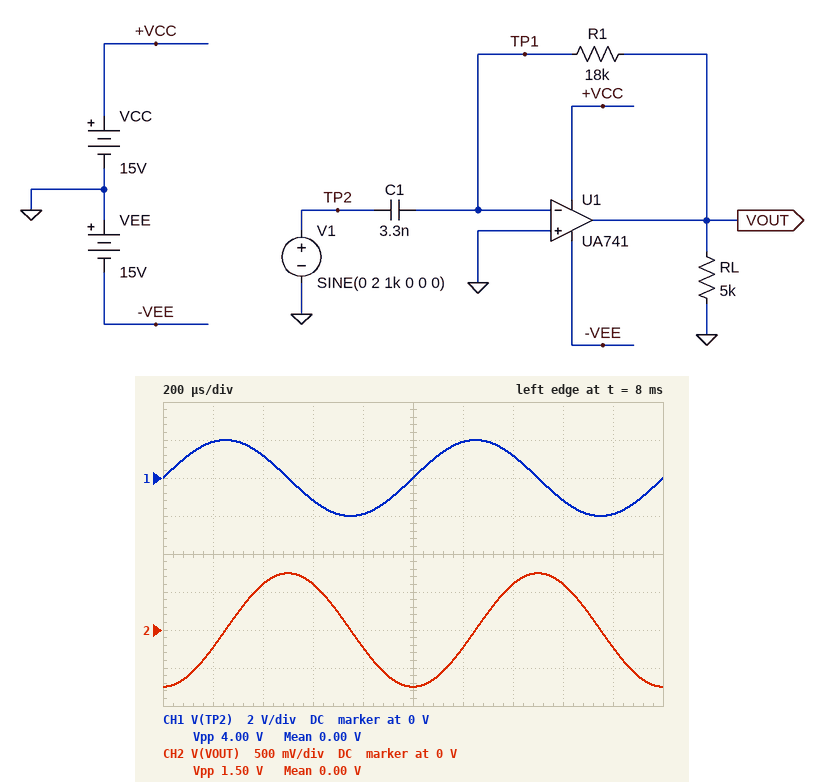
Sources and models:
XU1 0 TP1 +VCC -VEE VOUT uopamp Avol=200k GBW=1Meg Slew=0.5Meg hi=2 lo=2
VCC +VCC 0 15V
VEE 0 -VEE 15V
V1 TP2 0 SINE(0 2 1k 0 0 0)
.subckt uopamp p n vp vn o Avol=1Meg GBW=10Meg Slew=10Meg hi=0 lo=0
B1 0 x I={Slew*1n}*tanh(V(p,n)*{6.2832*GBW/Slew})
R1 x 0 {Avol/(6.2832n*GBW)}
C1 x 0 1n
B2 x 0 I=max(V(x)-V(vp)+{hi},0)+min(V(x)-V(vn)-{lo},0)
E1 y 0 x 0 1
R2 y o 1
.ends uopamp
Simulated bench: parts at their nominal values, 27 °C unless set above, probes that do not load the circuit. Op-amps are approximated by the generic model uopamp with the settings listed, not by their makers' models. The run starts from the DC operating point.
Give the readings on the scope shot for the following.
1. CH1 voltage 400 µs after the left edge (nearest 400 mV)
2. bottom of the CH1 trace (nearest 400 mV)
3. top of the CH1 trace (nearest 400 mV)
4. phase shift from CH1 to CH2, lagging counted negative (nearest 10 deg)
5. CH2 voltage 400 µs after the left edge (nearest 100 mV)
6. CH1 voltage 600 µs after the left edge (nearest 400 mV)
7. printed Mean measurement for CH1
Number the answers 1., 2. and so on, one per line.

1. 1.2 V
2. -2.0 V
3. 2.0 V
4. -90 deg
5. 600 mV
6. -1.2 V
7. 0.00 V
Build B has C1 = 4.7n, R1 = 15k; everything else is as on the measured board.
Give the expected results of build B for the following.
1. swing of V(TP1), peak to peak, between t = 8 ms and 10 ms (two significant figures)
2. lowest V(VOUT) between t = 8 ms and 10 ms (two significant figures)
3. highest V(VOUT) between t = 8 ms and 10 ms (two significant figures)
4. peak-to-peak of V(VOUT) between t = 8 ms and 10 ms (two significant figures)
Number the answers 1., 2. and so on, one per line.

1. 1.8 mV
2. -890 mV
3. 890 mV
4. 1.8 V
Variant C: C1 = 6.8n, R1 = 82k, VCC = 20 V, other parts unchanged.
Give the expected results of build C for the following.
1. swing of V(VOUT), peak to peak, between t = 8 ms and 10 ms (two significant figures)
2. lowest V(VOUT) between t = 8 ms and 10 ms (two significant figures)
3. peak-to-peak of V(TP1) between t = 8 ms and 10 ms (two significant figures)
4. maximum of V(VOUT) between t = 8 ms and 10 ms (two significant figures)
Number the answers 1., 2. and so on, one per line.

1. 14 V
2. -7.0 V
3. 14 mV
4. 7.0 V
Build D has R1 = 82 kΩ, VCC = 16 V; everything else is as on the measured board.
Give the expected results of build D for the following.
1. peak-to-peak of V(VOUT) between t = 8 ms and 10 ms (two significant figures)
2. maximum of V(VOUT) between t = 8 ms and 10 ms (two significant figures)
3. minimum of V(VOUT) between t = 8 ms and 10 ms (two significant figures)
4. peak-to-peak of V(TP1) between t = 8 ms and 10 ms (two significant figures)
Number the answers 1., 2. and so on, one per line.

1. 6.8 V
2. 3.4 V
3. -3.4 V
4. 6.8 mV
